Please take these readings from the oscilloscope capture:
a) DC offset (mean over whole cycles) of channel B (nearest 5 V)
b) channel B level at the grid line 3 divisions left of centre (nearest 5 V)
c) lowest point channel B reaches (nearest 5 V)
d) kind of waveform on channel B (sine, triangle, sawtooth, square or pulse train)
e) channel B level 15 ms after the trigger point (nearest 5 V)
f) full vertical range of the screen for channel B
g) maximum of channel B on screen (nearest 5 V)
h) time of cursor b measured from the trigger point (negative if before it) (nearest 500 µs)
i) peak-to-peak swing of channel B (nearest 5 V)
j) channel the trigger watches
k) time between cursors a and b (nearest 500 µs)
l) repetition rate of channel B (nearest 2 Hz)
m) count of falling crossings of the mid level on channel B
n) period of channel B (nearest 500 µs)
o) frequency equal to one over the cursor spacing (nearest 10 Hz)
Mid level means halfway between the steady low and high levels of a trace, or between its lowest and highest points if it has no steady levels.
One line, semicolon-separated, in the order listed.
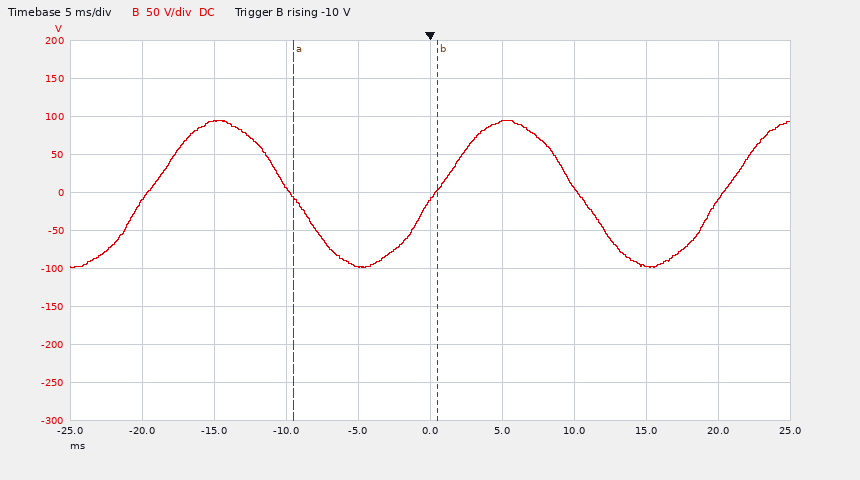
0 V; 95 V; -100 V; sine; -95 V; 500 V; 95 V; +500 µs; 195 V; channel B; 10.0 ms; 50 Hz; 2; 20.0 ms; 100 Hz
